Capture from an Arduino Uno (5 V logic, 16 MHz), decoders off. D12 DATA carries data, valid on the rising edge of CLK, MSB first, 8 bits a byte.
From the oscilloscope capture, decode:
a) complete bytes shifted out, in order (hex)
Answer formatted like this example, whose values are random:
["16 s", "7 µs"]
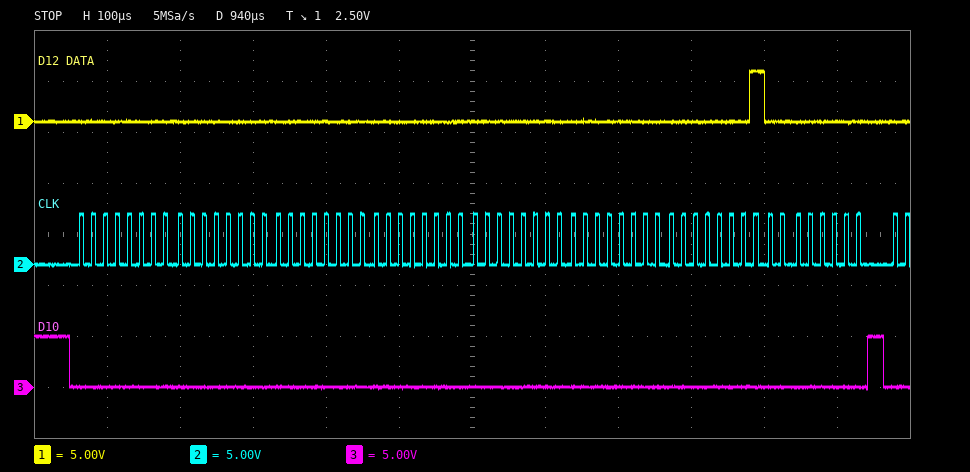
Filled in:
["00 00 00 00 00 00 01 00"]
